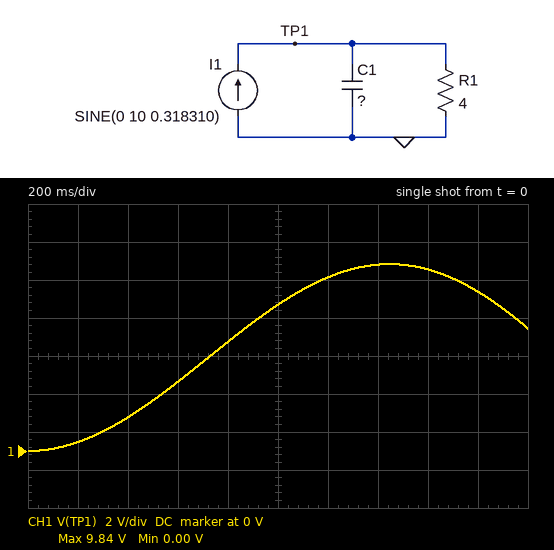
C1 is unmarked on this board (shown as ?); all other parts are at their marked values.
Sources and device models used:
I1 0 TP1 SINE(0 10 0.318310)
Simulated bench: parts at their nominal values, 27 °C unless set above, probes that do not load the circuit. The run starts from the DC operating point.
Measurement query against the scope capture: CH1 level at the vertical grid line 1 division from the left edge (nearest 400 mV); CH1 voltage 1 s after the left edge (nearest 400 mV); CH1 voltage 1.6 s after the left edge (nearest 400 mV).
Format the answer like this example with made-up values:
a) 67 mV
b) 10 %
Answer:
a) 400 mV
b) 7.6 V
c) 9.6 V
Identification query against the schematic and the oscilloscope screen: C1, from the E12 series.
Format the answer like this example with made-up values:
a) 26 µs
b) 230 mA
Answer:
a) 820 mF
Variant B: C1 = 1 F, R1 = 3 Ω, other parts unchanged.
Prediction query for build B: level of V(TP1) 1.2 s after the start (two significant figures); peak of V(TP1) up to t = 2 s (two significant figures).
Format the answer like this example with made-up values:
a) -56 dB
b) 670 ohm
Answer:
a) 7.4 V
b) 7.9 V
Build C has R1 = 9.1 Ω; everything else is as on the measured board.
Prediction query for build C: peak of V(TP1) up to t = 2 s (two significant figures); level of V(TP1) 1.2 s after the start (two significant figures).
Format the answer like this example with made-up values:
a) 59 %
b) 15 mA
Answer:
a) 11 V
b) 9.9 V
